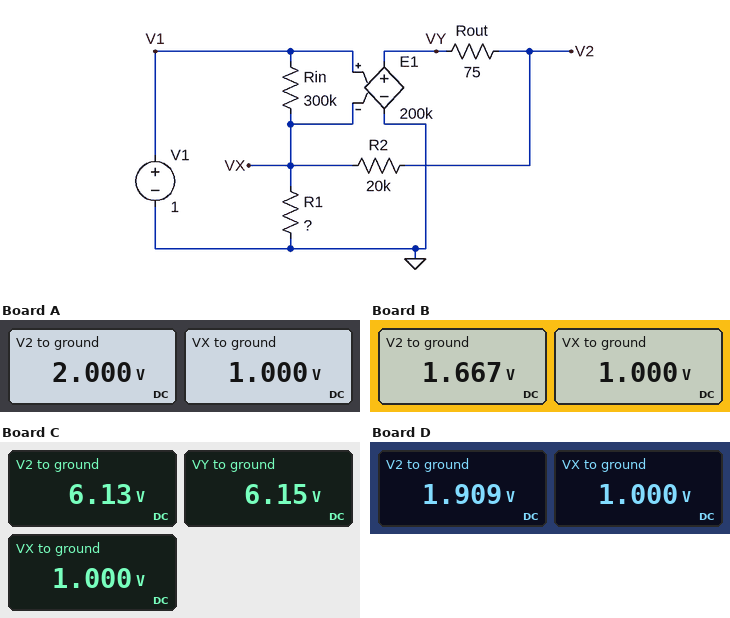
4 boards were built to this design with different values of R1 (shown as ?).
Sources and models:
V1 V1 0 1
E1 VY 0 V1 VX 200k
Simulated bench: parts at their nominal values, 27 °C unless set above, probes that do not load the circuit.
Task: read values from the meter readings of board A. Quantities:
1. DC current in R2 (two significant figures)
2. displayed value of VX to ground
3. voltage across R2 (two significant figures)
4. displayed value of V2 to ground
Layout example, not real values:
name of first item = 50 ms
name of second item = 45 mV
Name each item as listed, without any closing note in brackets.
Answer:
DC current in R2 = 50 µA
displayed value of VX to ground = 1.000 V
voltage across R2 = 1.0 V
displayed value of V2 to ground = 2.000 V
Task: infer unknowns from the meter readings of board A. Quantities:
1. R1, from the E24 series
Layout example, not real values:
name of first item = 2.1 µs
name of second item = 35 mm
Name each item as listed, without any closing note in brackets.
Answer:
R1, from the E24 series = 20 kΩ
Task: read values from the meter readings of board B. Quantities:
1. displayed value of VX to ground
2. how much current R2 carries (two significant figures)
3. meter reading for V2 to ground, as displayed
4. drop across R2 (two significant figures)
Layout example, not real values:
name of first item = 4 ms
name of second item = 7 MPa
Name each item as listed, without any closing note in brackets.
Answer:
displayed value of VX to ground = 1.000 V
how much current R2 carries = 33 µA
meter reading for V2 to ground, as displayed = 1.667 V
drop across R2 = 670 mV
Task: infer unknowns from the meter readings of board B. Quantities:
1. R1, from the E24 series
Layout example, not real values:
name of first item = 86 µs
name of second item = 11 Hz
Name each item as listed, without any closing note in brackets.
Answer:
R1, from the E24 series = 30 kΩ
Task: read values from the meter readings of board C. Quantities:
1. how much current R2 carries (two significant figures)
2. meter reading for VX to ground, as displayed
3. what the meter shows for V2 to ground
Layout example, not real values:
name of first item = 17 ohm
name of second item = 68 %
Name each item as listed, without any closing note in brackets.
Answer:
how much current R2 carries = 260 µA
meter reading for VX to ground, as displayed = 1.000 V
what the meter shows for V2 to ground = 6.13 V
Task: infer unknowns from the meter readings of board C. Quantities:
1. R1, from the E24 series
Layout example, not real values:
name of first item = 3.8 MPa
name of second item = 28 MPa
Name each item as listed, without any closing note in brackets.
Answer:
R1, from the E24 series = 3.9 kΩ
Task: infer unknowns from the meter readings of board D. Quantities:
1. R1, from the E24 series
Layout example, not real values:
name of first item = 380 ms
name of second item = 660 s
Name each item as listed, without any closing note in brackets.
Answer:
R1, from the E24 series = 22 kΩ
